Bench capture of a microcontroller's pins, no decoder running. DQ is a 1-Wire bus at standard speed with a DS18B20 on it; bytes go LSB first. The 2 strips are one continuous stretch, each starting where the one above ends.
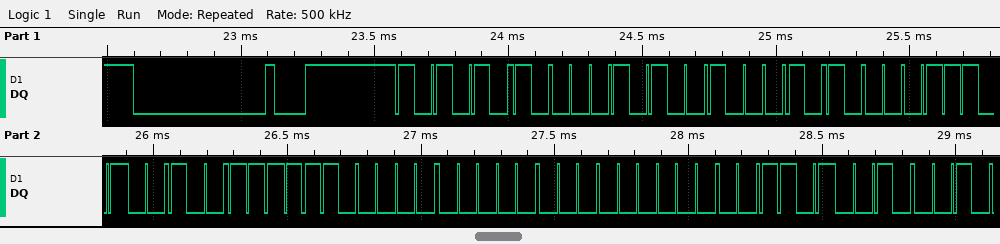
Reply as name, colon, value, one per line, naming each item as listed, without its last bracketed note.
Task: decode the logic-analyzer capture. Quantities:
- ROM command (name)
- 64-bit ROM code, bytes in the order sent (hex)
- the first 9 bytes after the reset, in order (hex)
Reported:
ROM command: Match ROM
64-bit ROM code, bytes in the order sent: 28 51 B8 E4 07 00 00 4B
the first 9 bytes after the reset, in order: 55 28 51 B8 E4 07 00 00 4B
